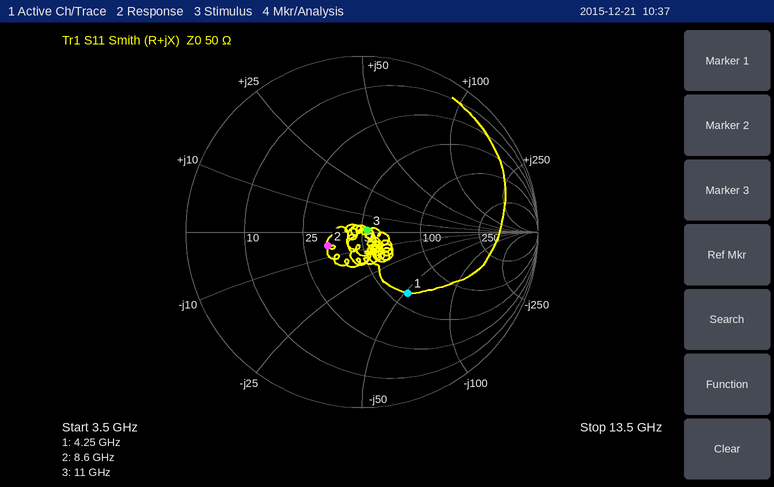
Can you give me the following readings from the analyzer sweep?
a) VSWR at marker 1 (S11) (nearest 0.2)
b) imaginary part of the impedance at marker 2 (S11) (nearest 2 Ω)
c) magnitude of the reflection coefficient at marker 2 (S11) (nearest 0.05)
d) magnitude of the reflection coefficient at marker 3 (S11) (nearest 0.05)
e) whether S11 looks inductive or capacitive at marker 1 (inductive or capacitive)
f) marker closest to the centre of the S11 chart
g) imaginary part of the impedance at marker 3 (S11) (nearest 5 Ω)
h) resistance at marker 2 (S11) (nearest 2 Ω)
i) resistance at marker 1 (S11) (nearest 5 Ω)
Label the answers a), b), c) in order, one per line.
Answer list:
a) 2.6
b) -6 Ω
c) 0.20
d) 0.05
e) capacitive
f) marker 3
g) 0 Ω
h) 34 Ω
i) 60 Ω
